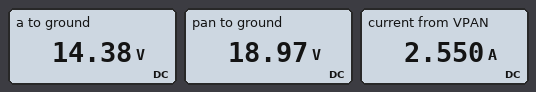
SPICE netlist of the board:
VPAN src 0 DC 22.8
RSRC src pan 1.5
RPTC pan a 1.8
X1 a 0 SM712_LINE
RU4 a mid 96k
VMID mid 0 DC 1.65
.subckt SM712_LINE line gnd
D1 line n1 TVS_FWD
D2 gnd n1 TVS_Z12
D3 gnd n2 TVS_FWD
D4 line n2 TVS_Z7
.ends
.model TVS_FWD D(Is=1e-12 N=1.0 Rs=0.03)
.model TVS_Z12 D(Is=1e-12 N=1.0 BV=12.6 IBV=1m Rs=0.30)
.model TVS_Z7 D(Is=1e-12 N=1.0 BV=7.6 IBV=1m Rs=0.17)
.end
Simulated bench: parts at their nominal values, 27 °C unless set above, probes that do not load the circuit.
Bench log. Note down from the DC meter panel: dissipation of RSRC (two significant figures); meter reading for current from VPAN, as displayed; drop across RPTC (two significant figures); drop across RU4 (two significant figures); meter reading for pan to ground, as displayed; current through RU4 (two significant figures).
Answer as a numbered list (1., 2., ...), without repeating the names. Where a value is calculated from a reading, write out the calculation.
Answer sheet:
1. (22.8 V - 18.97 V)^2 / 1.5 Ω = 9.8 W
2. 2.550 A
3. 18.97 V - 14.38 V = 4.6 V
4. 14.38 V - 1.65 V = 13 V
5. 18.97 V
6. (14.38 V - 1.65 V) / 96 kΩ = 130 µA
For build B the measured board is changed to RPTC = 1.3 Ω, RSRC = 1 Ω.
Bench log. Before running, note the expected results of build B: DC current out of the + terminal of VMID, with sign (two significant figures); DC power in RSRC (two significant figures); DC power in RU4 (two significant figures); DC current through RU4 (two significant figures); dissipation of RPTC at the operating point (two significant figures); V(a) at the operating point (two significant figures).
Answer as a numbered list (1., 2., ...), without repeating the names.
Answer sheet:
1. -140 µA
2. 12 W
3. 1.8 mW
4. 140 µA
5. 16 W
6. 15 V
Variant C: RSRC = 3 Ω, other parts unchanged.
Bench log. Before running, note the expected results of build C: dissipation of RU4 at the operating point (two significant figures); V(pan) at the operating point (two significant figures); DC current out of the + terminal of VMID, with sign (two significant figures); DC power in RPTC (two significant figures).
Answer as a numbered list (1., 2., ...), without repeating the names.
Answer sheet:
1. 1.6 mW
2. 17 V
3. -130 µA
4. 5.9 W
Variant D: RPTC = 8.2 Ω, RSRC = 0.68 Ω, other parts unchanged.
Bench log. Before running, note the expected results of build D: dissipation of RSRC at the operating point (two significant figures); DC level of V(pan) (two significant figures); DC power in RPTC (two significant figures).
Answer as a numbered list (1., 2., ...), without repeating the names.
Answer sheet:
1. 690 mW
2. 22 V
3. 8.4 W
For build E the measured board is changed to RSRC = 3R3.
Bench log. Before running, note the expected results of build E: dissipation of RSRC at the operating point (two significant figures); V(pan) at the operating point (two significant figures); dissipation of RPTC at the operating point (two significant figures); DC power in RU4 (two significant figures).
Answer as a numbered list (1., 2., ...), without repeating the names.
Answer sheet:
1. 9.6 W
2. 17 V
3. 5.3 W
4. 1.6 mW
